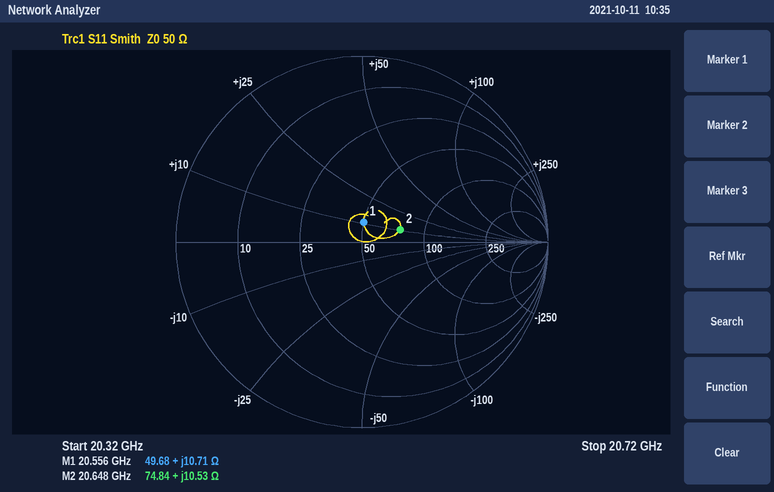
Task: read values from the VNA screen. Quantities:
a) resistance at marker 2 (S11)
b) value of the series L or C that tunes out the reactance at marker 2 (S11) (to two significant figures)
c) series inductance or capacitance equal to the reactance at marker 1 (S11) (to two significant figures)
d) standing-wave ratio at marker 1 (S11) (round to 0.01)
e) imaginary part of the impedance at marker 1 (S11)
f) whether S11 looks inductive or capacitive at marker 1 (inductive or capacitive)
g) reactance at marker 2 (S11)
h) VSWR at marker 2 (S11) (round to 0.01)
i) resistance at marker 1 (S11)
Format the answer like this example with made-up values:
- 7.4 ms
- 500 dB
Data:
- 74.84 Ω
- 730 fF
- 83 pH
- 1.24
- +10.71 Ω
- inductive
- +10.53 Ω
- 1.55
- 49.68 Ω
